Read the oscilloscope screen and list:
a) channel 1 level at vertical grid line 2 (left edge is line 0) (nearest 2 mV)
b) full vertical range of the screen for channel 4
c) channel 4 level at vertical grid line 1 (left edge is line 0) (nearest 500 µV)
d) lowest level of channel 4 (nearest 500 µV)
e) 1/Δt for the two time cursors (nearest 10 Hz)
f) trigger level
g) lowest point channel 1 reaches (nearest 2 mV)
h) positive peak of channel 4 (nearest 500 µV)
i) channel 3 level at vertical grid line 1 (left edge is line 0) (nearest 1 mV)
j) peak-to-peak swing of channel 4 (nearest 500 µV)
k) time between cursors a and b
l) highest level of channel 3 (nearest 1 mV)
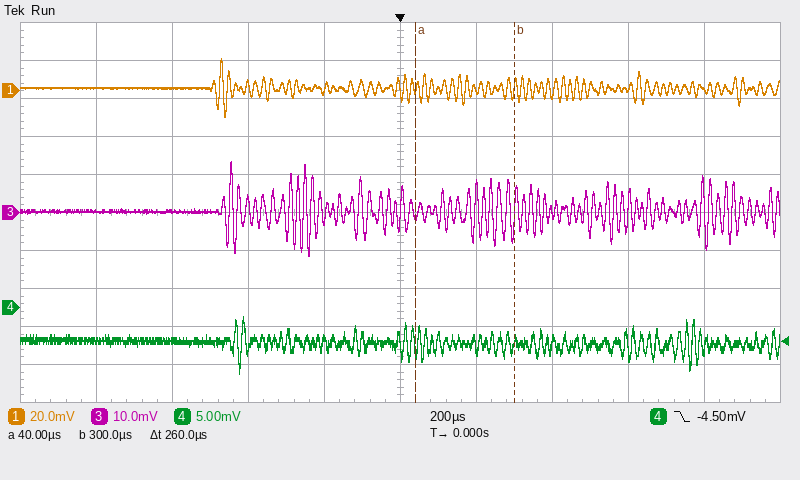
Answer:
2 mV
50 mV
-4.5 mV
-8.5 mV
3.85 kHz
-4.50 mV
-14 mV
-1.0 mV
0 mV
7.5 mV
260 µs
13 mV
